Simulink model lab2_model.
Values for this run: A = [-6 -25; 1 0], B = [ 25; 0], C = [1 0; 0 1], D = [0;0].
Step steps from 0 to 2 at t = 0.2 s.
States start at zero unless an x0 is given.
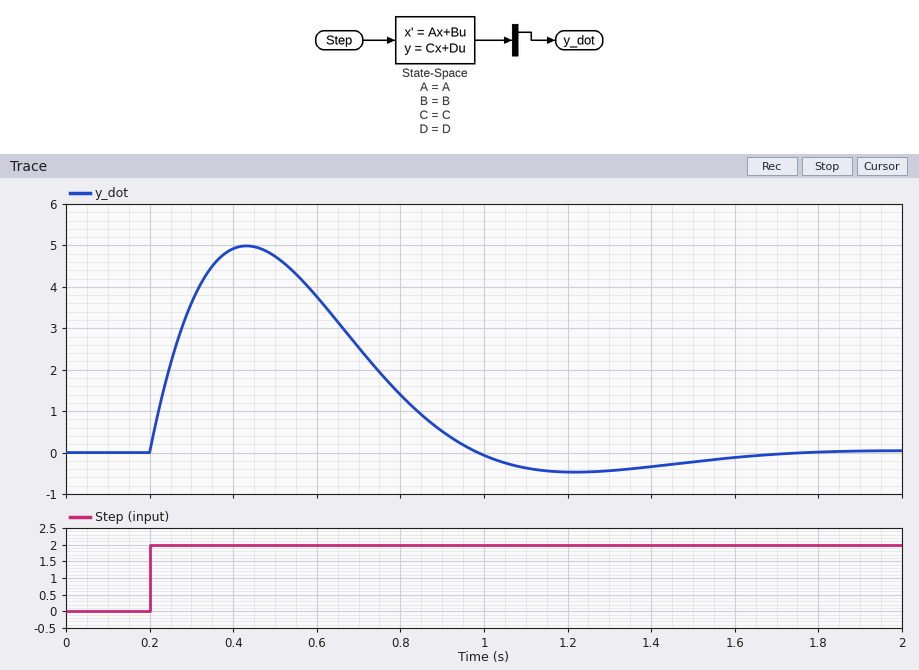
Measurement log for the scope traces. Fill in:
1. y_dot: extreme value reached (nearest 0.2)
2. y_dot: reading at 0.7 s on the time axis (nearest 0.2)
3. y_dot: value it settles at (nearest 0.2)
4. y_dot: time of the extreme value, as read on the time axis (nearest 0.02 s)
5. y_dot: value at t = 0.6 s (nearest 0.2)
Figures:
5.0
2.6
0.0
0.44 s
3.8
